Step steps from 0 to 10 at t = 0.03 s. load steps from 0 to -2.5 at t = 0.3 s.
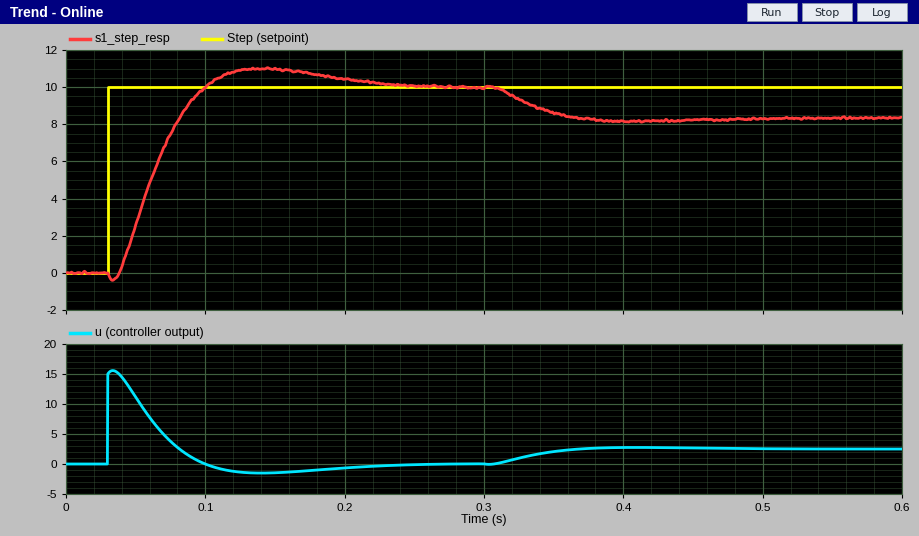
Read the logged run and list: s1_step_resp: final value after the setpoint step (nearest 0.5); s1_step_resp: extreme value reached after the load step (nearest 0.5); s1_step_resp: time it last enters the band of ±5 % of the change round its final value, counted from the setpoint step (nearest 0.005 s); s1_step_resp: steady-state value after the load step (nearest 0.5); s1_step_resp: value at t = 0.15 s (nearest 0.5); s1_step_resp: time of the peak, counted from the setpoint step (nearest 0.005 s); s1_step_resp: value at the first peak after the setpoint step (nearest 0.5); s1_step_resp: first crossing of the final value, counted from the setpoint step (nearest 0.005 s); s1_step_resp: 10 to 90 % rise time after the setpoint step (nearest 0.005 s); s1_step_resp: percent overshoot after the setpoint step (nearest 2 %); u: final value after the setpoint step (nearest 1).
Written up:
10.0
8.0
0.165 s
8.5
11.0
0.110 s
11.0
0.070 s
0.045 s
10 %
0
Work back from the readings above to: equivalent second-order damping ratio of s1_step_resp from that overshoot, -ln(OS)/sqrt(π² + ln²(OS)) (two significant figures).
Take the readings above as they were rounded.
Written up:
0.59
